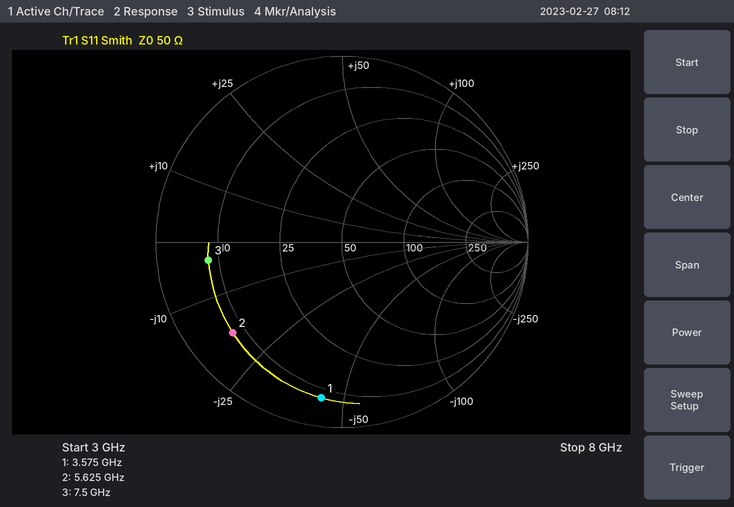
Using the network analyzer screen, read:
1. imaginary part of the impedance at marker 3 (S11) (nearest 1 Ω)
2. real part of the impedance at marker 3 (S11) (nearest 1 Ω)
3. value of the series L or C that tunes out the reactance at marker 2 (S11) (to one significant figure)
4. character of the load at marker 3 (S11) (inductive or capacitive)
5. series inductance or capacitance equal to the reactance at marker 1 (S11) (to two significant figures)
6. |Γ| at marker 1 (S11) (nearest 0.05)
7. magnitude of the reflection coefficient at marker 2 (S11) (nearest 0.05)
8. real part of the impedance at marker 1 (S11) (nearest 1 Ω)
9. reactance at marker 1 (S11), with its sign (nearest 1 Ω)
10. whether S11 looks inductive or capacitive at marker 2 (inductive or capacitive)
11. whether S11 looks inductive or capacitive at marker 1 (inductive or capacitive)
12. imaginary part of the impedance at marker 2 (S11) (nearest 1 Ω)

-3 Ω
8 Ω
500 pH
capacitive
1.0 pF
0.85
0.75
7 Ω
-43 Ω
capacitive
capacitive
-18 Ω
